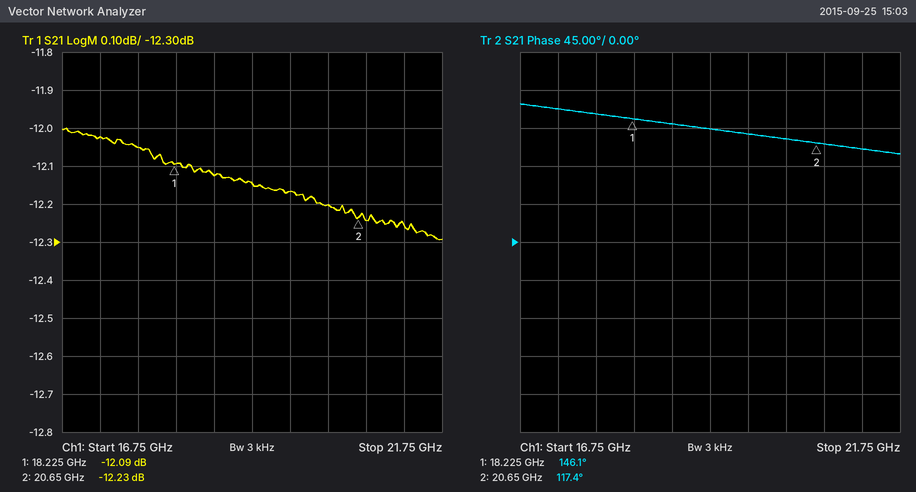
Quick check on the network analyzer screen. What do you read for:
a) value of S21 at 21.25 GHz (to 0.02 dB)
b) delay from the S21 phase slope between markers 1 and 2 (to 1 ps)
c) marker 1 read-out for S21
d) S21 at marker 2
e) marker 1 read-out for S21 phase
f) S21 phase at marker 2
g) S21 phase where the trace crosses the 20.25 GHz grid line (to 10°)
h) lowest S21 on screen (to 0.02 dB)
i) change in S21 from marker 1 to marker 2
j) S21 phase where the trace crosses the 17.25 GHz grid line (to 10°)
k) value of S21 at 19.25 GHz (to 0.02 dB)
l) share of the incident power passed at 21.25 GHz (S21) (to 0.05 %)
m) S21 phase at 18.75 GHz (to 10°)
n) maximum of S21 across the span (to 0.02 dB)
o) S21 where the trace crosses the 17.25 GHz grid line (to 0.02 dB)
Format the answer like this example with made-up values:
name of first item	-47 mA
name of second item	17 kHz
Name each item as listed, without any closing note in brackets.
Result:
value of S21 at 21.25 GHz	-12.26 dB
delay from the S21 phase slope between markers 1 and 2	33 ps
marker 1 read-out for S21	-12.09 dB
S21 at marker 2	-12.23 dB
marker 1 read-out for S21 phase	146.1°
S21 phase at marker 2	117.4°
S21 phase where the trace crosses the 20.25 GHz grid line	120°
lowest S21 on screen	-12.30 dB
change in S21 from marker 1 to marker 2	-0.14 dB
S21 phase where the trace crosses the 17.25 GHz grid line	160°
value of S21 at 19.25 GHz	-12.14 dB
share of the incident power passed at 21.25 GHz (S21)	5.95 %
S21 phase at 18.75 GHz	140°
maximum of S21 across the span	-12.00 dB
S21 where the trace crosses the 17.25 GHz grid line	-12.02 dB
